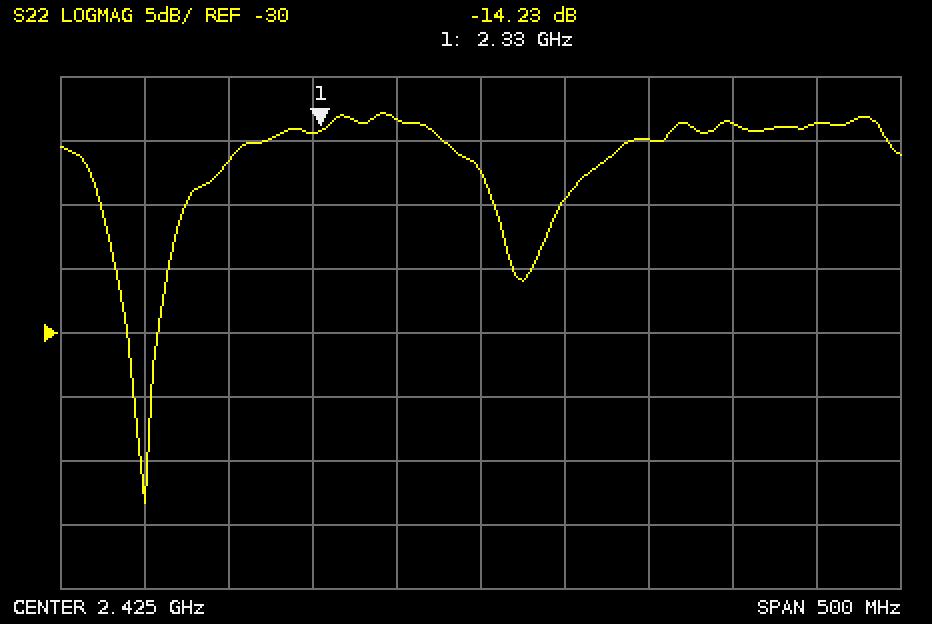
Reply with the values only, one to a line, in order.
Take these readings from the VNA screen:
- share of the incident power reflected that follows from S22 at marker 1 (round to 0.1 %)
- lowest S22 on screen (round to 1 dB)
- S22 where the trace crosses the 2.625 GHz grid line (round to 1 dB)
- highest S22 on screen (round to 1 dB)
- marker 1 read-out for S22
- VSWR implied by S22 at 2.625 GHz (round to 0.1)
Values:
3.8 %
-43 dB
-14 dB
-13 dB
-14.23 dB
1.5
